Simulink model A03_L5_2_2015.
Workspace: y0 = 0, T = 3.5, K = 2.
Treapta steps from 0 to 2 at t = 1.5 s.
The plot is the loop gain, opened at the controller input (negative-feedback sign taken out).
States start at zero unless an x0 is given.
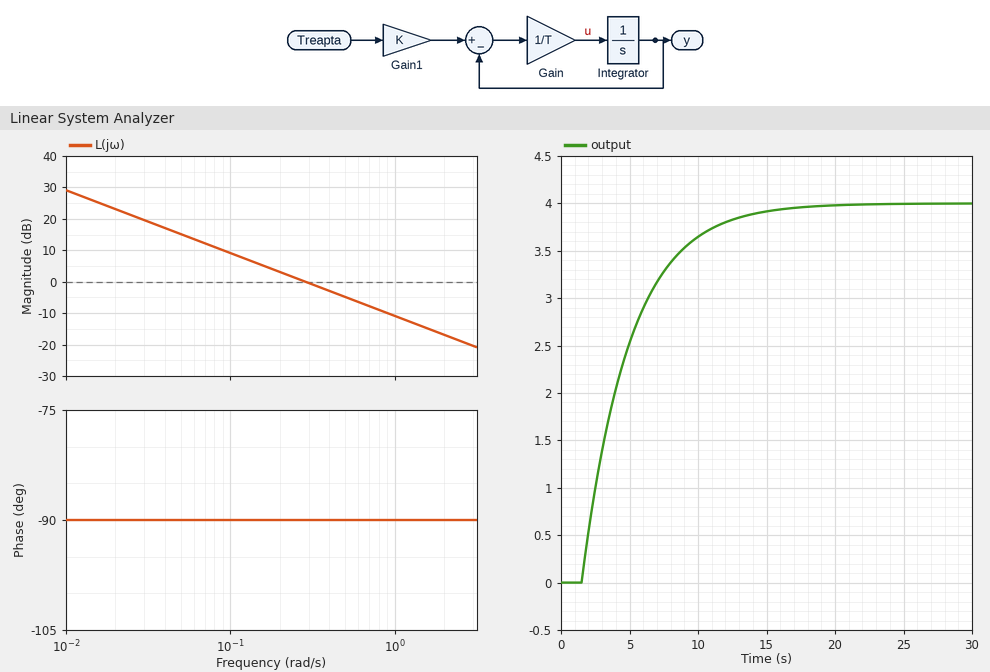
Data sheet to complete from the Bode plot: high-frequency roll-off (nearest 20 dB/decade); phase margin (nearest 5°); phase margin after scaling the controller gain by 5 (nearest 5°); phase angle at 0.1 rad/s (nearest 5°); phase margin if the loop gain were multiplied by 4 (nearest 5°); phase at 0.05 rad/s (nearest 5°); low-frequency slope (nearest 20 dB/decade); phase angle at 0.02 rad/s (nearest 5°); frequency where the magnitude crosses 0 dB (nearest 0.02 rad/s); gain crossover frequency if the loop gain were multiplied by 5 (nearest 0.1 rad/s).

-20 dB/decade
90°
90°
-90°
90°
-90°
-20 dB/decade
-90°
0.28 rad/s
1.4 rad/s
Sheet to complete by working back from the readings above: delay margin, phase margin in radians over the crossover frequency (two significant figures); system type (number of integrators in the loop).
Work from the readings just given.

5.6 s
1
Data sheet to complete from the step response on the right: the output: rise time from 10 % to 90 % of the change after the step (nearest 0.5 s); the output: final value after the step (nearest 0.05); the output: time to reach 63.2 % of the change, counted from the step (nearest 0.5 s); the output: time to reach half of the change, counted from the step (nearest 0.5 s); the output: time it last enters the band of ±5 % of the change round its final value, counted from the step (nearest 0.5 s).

7.5 s
4.00
3.5 s
2.5 s
10.5 s
